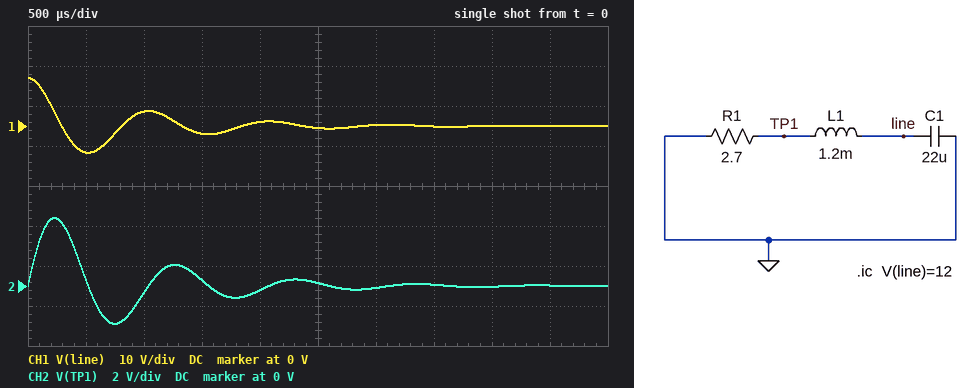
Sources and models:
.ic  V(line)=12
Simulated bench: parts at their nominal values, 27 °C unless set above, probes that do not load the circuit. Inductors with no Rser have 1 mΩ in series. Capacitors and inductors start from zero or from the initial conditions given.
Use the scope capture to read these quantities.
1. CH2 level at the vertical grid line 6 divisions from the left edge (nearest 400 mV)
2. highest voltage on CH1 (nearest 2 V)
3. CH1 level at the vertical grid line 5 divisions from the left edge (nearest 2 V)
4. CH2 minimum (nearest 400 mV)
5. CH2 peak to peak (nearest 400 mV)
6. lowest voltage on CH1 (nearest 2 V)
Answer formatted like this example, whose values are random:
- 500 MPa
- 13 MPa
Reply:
- 0 V
- 12 V
- 0 V
- -2.0 V
- 5.2 V
- -6 V
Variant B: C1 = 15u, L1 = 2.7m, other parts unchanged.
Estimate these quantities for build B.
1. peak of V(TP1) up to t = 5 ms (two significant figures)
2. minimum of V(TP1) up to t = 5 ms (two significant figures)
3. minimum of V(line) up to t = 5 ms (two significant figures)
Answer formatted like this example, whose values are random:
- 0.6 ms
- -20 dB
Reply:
- 2.1 V
- -1.5 V
- -8.7 V
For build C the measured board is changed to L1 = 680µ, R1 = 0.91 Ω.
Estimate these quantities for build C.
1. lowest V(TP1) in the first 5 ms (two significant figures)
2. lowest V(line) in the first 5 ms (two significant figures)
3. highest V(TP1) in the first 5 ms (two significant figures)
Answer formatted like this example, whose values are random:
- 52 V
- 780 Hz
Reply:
- -1.3 V
- -9.3 V
- 1.7 V
